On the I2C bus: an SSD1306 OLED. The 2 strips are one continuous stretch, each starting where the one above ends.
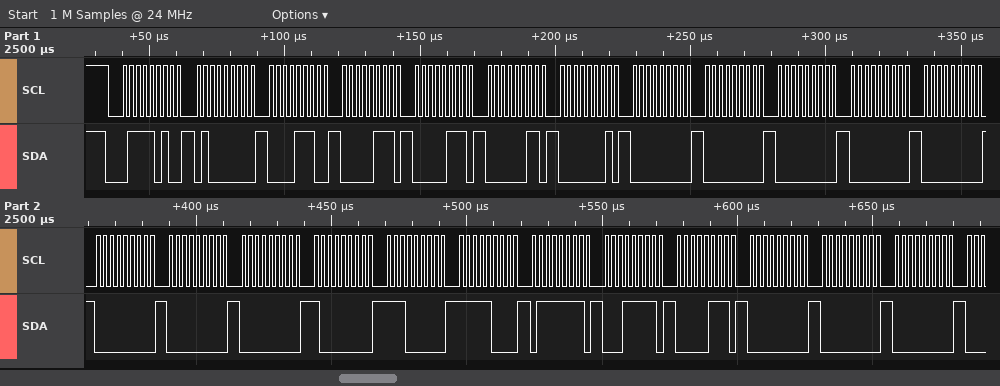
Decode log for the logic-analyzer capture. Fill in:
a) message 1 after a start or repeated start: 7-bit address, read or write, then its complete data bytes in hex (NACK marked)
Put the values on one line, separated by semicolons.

0x3D write: 40 0E 07 07 03 01 00 00 00 00 00 00 00 00 80 E0 F8 7F 1F 07 00 00 00
